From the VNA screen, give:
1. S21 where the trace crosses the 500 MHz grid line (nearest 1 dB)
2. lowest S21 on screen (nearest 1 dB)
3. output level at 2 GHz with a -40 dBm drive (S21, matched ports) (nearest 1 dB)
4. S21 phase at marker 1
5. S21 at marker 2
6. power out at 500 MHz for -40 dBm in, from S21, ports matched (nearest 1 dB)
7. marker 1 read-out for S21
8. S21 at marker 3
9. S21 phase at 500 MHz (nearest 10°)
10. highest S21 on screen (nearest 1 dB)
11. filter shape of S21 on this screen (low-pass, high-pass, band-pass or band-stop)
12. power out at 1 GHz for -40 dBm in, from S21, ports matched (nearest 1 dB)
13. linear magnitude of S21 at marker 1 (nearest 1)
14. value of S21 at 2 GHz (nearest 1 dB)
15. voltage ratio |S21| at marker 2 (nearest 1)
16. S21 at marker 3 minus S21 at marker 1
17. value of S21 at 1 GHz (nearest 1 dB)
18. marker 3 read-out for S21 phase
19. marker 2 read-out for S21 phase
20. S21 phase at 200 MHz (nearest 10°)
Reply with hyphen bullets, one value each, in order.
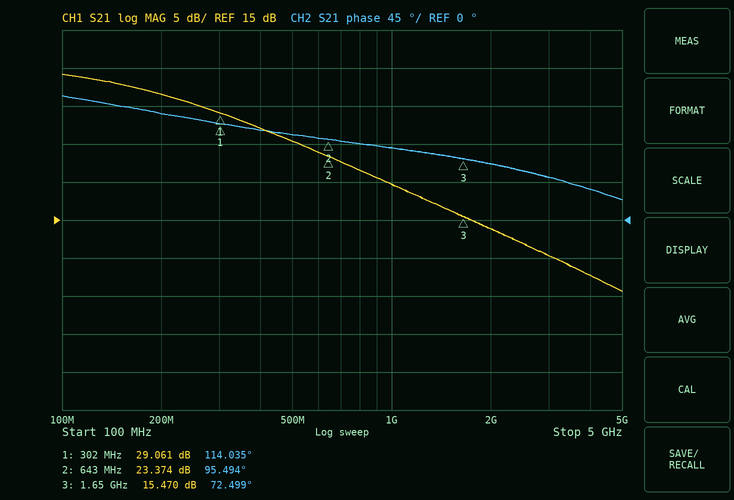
- 25 dB
- 6 dB
- -26 dBm
- 114.035°
- 23.374 dB
- -15 dBm
- 29.061 dB
- 15.470 dB
- 100°
- 34 dB
- low-pass
- -20 dBm
- 28
- 14 dB
- 15
- -13.591 dB
- 20 dB
- 72.499°
- 95.494°
- 130°
